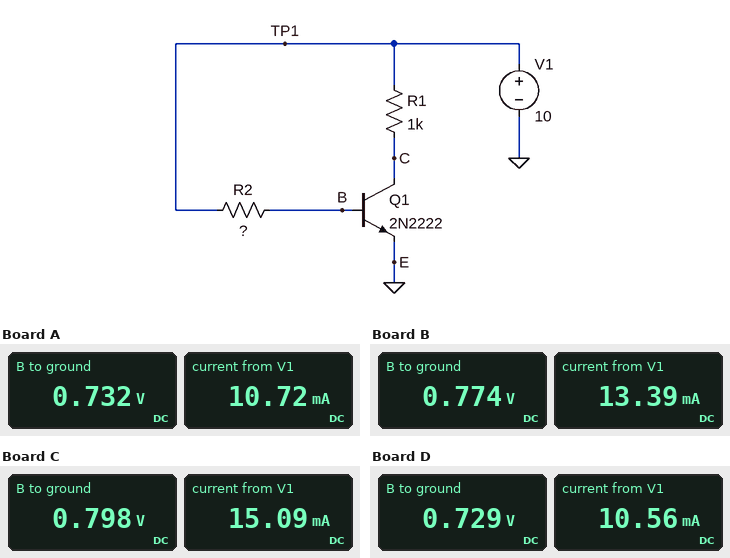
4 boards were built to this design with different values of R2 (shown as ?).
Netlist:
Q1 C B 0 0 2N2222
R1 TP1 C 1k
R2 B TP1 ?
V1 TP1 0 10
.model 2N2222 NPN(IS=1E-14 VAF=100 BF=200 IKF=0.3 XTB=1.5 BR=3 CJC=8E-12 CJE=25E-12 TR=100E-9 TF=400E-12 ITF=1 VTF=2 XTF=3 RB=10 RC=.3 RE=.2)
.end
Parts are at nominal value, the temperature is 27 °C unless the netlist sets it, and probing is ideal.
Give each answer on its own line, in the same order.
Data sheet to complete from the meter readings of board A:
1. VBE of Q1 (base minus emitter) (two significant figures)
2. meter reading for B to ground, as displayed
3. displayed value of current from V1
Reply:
730 mV
0.732 V
10.72 mA
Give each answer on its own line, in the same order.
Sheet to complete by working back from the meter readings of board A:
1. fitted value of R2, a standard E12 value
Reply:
12 kΩ
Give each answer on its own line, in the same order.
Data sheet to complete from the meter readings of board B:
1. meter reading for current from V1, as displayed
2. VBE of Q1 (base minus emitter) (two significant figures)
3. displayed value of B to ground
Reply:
13.39 mA
770 mV
0.774 V
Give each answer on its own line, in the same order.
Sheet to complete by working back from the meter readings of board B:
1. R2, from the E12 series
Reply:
2.7 kΩ
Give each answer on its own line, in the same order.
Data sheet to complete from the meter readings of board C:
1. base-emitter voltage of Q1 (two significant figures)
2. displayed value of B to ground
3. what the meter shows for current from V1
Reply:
800 mV
0.798 V
15.09 mA
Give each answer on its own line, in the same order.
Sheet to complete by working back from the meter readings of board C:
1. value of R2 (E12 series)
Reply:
1.8 kΩ
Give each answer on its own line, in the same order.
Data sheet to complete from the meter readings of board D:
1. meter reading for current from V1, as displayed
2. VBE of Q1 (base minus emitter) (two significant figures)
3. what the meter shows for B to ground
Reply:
10.56 mA
730 mV
0.729 V
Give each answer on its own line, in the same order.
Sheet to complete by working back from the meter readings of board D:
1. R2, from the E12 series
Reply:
15 kΩ
